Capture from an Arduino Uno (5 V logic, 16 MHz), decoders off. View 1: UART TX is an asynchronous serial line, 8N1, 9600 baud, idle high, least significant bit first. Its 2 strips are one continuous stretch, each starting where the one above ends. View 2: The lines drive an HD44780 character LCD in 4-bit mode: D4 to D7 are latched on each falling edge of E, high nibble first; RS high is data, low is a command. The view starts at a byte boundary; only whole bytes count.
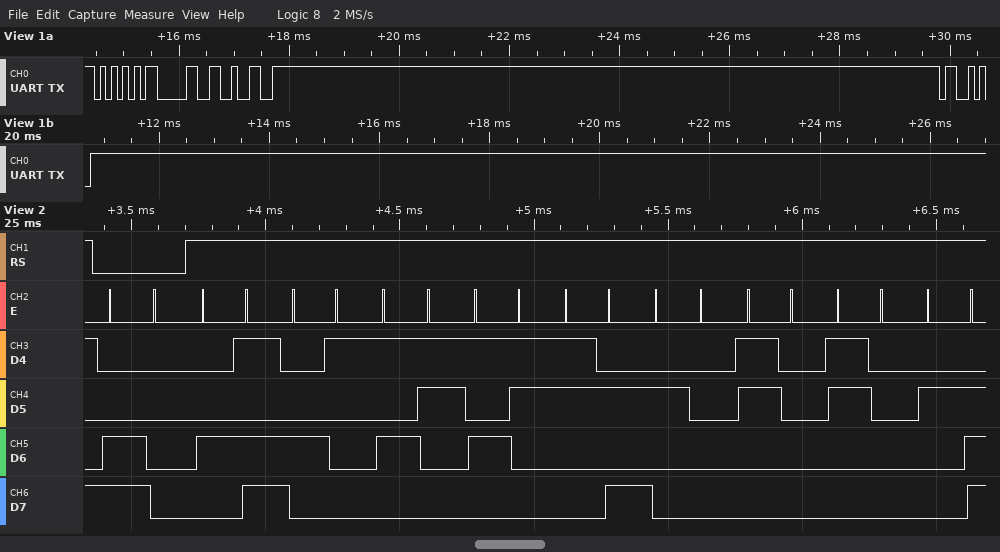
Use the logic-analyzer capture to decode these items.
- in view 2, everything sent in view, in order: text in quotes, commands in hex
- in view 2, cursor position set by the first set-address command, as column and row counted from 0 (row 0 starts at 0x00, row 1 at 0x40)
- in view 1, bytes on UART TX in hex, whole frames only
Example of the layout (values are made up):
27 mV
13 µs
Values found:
0xC0 "MASS: 00."
column 0, row 1
55 30 32 53
